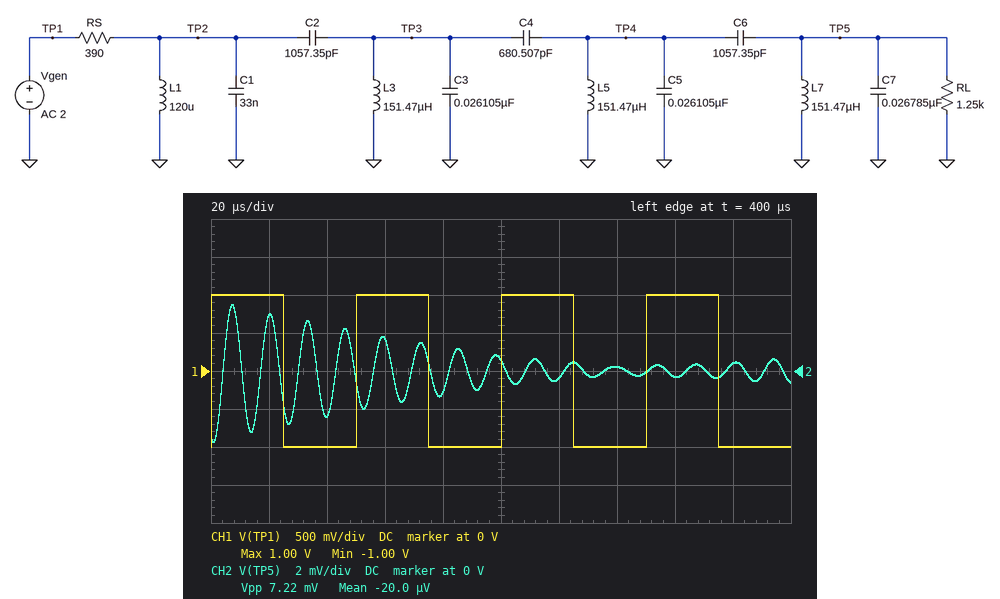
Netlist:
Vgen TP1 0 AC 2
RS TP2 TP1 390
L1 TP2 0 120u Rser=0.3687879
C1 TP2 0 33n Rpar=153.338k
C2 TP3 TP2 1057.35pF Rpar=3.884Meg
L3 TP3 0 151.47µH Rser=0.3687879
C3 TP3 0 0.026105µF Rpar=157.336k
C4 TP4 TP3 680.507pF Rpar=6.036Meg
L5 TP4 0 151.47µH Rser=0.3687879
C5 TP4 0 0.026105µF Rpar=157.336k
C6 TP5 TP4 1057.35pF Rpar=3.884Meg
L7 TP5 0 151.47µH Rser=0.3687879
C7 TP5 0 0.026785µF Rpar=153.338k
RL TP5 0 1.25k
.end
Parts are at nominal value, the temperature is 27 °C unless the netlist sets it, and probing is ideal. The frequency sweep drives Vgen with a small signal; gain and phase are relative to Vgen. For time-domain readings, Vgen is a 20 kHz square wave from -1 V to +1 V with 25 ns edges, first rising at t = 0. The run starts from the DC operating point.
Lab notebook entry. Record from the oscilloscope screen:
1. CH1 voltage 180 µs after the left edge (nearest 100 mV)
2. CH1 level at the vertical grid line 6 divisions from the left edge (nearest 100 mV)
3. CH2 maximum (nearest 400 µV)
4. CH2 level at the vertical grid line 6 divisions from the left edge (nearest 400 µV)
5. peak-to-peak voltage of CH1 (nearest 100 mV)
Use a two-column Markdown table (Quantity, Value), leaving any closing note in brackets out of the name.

| Quantity | Value |
|---|---|
| CH1 voltage 180 µs after the left edge | -1.0 V |
| CH1 level at the vertical grid line 6 divisions from the left edge | 1.0 V |
| CH2 maximum | 3.6 mV |
| CH2 level at the vertical grid line 6 divisions from the left edge | -400 µV |
| peak-to-peak voltage of CH1 | 2.0 V |
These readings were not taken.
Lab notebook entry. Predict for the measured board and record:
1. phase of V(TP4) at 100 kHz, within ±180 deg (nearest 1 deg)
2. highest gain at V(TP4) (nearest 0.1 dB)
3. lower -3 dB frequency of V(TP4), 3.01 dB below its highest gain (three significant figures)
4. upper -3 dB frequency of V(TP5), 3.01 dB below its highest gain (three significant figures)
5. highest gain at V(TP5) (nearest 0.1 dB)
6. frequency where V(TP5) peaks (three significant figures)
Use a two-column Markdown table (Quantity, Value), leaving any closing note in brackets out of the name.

| Quantity | Value |
|---|---|
| phase of V(TP4) at 100 kHz, within ±180 deg | -71 deg |
| highest gain at V(TP4) | -0.6 dB |
| lower -3 dB frequency of V(TP4), 3.01 dB below its highest gain | 76.0 kHz |
| upper -3 dB frequency of V(TP5), 3.01 dB below its highest gain | 79.0 kHz |
| highest gain at V(TP5) | -5.3 dB |
| frequency where V(TP5) peaks | 77.7 kHz |
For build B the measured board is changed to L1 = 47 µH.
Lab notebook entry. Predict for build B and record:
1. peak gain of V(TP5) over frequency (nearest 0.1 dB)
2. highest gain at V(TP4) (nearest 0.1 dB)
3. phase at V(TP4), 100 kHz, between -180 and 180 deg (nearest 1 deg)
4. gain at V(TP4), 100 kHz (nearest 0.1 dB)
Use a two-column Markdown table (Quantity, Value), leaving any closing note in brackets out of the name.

| Quantity | Value |
|---|---|
| peak gain of V(TP5) over frequency | -23.3 dB |
| highest gain at V(TP4) | -18.6 dB |
| phase at V(TP4), 100 kHz, between -180 and 180 deg | 77 deg |
| gain at V(TP4), 100 kHz | -58.6 dB |
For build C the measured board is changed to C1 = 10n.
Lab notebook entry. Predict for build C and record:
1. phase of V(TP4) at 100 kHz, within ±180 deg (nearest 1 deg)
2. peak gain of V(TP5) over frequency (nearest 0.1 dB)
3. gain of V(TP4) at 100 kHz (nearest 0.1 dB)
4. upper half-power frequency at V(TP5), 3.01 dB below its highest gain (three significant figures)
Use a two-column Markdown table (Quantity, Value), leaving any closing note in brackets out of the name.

| Quantity | Value |
|---|---|
| phase of V(TP4) at 100 kHz, within ±180 deg | 68 deg |
| peak gain of V(TP5) over frequency | -16.3 dB |
| gain of V(TP4) at 100 kHz | -53.2 dB |
| upper half-power frequency at V(TP5), 3.01 dB below its highest gain | 78.9 kHz |
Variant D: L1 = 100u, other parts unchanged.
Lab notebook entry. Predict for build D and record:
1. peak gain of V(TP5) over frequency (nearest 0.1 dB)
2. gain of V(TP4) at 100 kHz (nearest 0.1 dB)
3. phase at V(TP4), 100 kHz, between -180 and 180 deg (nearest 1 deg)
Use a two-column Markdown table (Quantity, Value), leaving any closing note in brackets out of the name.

| Quantity | Value |
|---|---|
| peak gain of V(TP5) over frequency | -8.9 dB |
| gain of V(TP4) at 100 kHz | -52.0 dB |
| phase at V(TP4), 100 kHz, between -180 and 180 deg | -63 deg |
